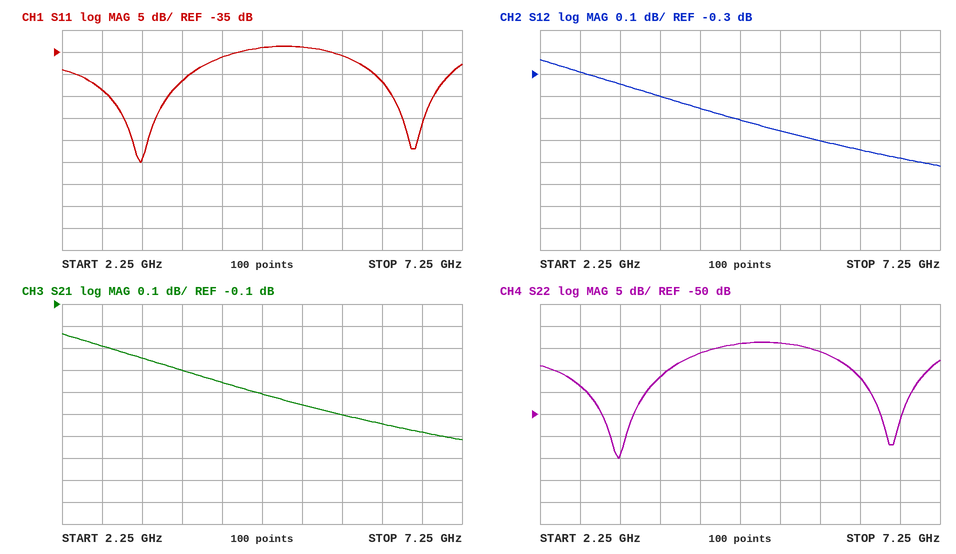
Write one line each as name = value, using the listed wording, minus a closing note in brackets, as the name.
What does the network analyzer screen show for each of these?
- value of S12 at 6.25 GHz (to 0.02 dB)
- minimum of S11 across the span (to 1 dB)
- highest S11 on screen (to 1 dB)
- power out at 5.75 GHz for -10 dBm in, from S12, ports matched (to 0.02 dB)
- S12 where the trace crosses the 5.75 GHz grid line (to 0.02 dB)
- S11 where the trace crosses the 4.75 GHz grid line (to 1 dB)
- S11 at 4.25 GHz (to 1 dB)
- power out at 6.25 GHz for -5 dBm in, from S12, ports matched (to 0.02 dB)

value of S12 at 6.25 GHz = -0.64 dB
minimum of S11 across the span = -60 dB
highest S11 on screen = -34 dB
power out at 5.75 GHz for -10 dBm in, from S12, ports matched = -10.60 dBm
S12 where the trace crosses the 5.75 GHz grid line = -0.60 dB
S11 where the trace crosses the 4.75 GHz grid line = -34 dB
S11 at 4.25 GHz = -36 dB
power out at 6.25 GHz for -5 dBm in, from S12, ports matched = -5.64 dBm
